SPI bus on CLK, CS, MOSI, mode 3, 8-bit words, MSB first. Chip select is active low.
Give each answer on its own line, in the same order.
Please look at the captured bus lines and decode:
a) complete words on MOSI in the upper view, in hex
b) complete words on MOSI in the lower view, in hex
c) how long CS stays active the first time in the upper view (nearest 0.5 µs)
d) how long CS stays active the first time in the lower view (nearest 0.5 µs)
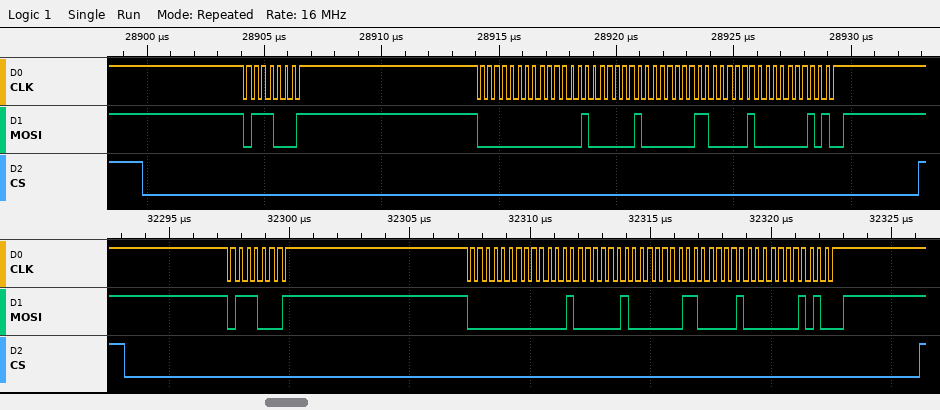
71, 00, 02, 04, 06, 08, 0A
71, 00, 04, 08, 0C, 10, 14
33 µs
33 µs
